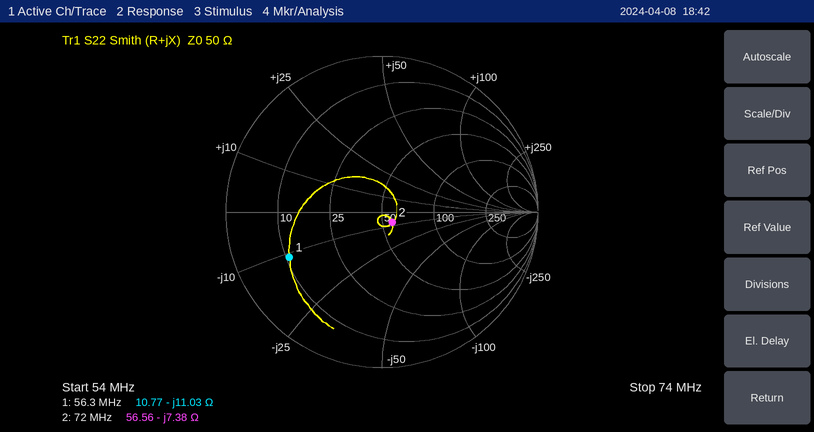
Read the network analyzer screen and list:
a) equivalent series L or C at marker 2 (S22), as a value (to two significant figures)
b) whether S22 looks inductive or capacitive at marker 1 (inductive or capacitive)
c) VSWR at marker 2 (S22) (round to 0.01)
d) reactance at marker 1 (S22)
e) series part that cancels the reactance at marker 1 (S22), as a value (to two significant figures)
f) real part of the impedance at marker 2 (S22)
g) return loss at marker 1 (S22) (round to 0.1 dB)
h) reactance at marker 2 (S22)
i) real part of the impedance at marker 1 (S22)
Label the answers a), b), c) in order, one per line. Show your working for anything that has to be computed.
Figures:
a) C = 1/(2π × 72 MHz × 7.38 Ω) ≈ 300 pF
b) capacitive
c) 1.20
d) -11.03 Ω
e) L = 11.03 Ω/(2π × 56.3 MHz) ≈ 31 nH
f) 56.56 Ω
g) 3.6 dB
h) -7.38 Ω
i) 10.77 Ω
